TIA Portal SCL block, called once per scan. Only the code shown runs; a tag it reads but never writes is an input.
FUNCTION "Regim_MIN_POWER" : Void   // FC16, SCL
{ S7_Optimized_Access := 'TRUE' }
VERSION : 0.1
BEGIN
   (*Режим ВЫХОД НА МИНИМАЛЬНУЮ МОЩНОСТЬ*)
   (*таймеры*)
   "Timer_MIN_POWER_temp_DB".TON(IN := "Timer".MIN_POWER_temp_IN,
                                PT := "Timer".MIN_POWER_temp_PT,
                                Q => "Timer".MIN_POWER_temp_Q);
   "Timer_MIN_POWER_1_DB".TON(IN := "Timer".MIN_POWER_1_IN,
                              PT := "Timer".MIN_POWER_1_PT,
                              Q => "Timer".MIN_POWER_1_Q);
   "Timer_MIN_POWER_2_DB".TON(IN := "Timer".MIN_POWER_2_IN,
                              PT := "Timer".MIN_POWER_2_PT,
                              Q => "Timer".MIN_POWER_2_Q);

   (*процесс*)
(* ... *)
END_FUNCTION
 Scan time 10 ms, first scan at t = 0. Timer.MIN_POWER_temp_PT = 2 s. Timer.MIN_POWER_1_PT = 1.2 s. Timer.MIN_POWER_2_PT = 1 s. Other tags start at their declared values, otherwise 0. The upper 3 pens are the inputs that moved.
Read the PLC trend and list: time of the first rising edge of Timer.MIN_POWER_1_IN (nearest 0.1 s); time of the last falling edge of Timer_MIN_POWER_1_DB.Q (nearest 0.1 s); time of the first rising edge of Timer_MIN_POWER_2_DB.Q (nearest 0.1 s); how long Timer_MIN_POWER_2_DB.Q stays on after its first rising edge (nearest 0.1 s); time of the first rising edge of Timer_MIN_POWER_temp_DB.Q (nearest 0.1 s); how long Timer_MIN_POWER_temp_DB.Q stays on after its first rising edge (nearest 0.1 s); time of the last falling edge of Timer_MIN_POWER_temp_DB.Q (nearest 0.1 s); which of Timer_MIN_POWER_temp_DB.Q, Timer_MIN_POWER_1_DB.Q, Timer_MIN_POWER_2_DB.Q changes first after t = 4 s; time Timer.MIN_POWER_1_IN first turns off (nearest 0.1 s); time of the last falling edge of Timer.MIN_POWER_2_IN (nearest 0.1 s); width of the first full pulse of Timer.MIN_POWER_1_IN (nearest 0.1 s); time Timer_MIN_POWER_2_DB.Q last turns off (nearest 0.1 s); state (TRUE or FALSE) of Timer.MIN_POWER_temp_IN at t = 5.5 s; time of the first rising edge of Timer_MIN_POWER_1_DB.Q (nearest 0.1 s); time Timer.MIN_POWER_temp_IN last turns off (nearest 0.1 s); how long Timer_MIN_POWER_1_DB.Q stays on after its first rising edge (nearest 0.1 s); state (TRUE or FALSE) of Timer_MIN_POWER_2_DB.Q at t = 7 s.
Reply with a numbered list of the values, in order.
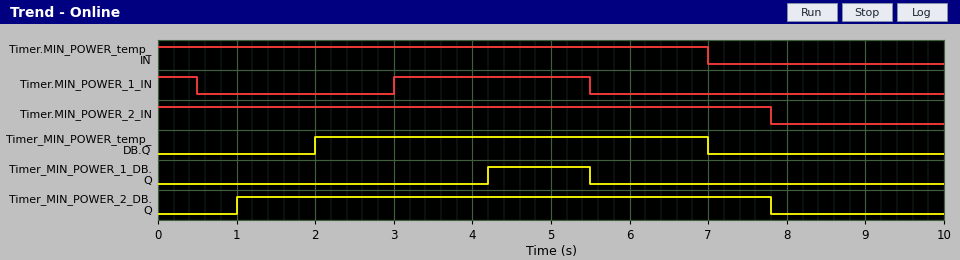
1. 3.0 s
2. 5.5 s
3. 1.0 s
4. 6.8 s
5. 2.0 s
6. 5.0 s
7. 7.0 s
8. Timer_MIN_POWER_1_DB.Q
9. 0.5 s
10. 7.8 s
11. 2.5 s
12. 7.8 s
13. TRUE
14. 4.2 s
15. 7.0 s
16. 1.3 s
17. TRUE
